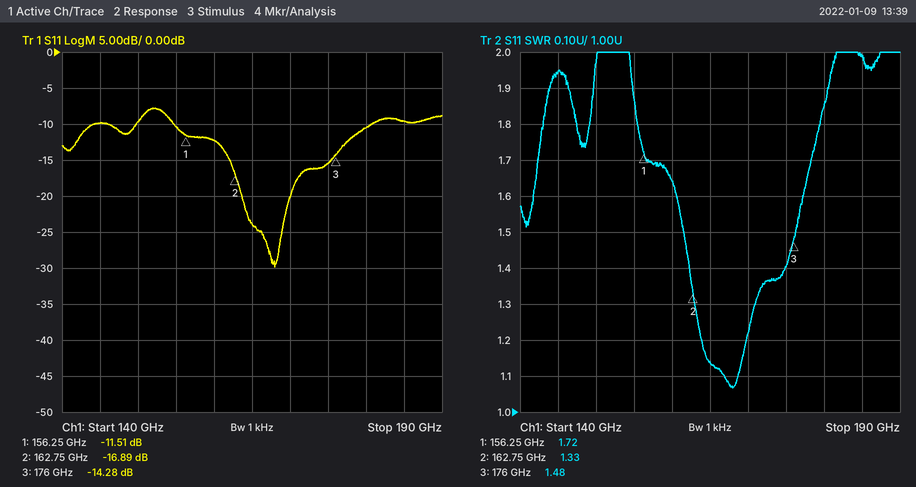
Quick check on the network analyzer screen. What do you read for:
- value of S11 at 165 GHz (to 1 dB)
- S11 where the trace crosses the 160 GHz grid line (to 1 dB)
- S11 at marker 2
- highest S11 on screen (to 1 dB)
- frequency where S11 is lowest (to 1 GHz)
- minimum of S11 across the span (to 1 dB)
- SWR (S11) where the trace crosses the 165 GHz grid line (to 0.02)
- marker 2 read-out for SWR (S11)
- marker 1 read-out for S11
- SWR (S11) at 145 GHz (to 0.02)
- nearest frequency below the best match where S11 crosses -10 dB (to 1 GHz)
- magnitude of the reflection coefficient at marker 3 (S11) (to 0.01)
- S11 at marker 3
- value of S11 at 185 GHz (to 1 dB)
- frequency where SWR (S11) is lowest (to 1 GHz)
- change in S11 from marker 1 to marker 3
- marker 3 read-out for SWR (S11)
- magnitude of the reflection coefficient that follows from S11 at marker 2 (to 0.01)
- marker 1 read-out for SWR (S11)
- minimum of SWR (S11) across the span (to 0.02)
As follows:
-24 dB
-12 dB
-16.89 dB
-8 dB
168 GHz
-30 dB
1.14
1.33
-11.51 dB
1.94
155 GHz
0.19
-14.28 dB
-10 dB
168 GHz
-2.77 dB
1.48
0.14
1.72
1.06
